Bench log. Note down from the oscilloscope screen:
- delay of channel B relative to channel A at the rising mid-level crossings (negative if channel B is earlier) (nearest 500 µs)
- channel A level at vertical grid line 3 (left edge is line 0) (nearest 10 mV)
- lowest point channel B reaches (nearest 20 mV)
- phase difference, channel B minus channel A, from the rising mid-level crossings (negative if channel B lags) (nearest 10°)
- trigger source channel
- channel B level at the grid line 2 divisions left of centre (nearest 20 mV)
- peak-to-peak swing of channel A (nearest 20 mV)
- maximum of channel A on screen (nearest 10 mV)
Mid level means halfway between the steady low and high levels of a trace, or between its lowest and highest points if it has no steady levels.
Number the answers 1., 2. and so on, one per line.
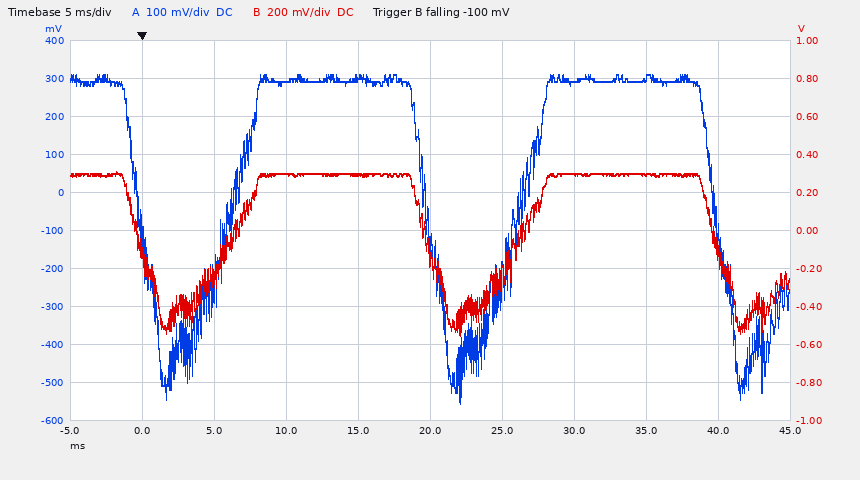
1. 0.0 ms
2. 290 mV
3. -560 mV
4. 0°
5. channel B
6. 300 mV
7. 860 mV
8. 310 mV
